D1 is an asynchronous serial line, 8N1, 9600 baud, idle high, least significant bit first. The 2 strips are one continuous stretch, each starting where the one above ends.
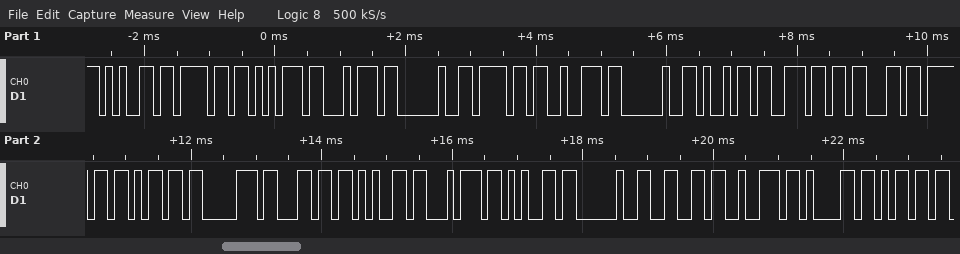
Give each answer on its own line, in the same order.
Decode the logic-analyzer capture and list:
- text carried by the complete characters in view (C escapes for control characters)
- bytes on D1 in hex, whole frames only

"eout or incomplete fram"
65 6F 75 74 20 6F 72 20 69 6E 63 6F 6D 70 6C 65 74 65 20 66 72 61 6D
